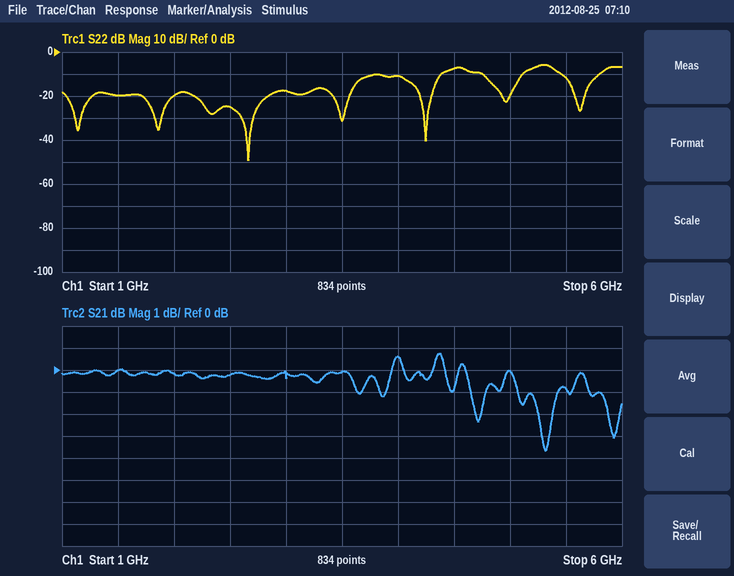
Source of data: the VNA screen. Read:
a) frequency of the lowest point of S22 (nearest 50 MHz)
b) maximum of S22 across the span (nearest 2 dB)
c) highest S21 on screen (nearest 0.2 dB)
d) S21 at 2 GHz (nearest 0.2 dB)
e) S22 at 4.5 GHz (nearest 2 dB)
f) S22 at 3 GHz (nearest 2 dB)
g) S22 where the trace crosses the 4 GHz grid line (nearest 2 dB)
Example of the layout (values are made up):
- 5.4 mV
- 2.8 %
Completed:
- 2.65 GHz
- -6 dB
- 0.8 dB
- -0.2 dB
- -8 dB
- -18 dB
- -10 dB
